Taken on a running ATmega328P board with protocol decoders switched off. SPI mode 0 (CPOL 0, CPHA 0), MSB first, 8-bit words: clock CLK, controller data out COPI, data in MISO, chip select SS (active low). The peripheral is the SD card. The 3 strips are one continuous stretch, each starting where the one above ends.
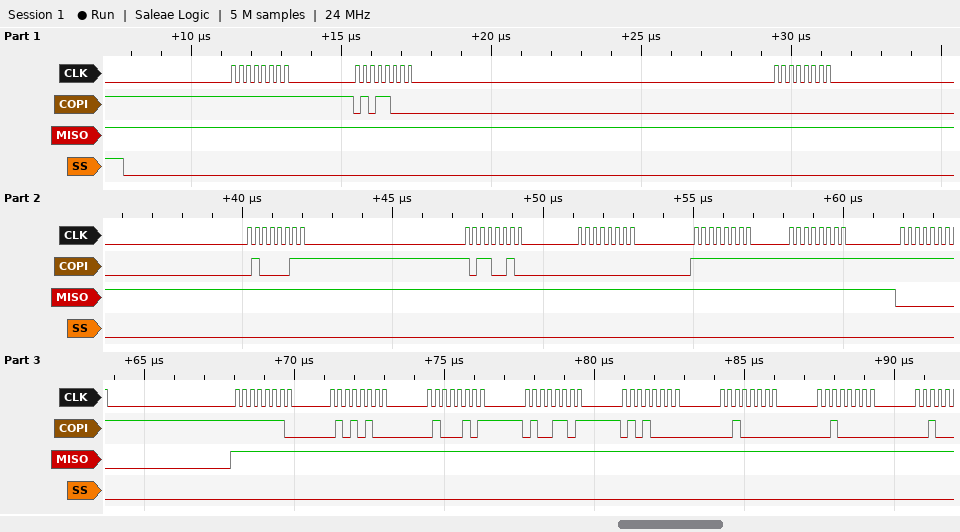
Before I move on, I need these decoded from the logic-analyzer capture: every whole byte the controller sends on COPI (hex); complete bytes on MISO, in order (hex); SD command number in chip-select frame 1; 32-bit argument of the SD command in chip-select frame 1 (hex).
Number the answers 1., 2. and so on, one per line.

1. 0xFF 0x58 0x00 0x43 0xB2 0x00 0xFF 0xFF 0xFF 0xFE 0x54 0x45 0x4D 0x50 0x20 0x20
2. 0xFF 0xFF 0xFF 0xFF 0xFF 0xFF 0xFF 0xFF 0x00 0xFF 0xFF 0xFF 0xFF 0xFF 0xFF 0xFF
3. CMD24
4. 0x0043B200
